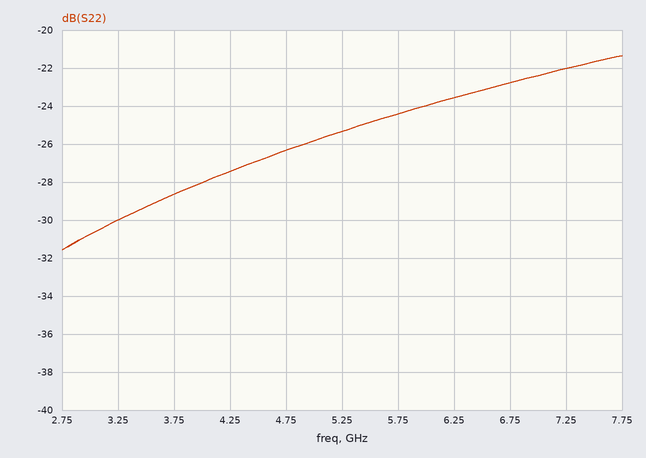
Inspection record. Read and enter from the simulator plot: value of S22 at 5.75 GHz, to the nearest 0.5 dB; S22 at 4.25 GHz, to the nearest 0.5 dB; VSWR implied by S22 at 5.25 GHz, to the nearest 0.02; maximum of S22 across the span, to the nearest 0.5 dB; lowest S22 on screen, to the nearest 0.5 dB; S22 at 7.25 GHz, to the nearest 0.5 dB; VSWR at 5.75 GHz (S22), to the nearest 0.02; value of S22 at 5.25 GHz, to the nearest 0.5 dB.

-24.5 dB
-27.5 dB
1.12
-21.5 dB
-31.5 dB
-22.0 dB
1.12
-25.5 dB
